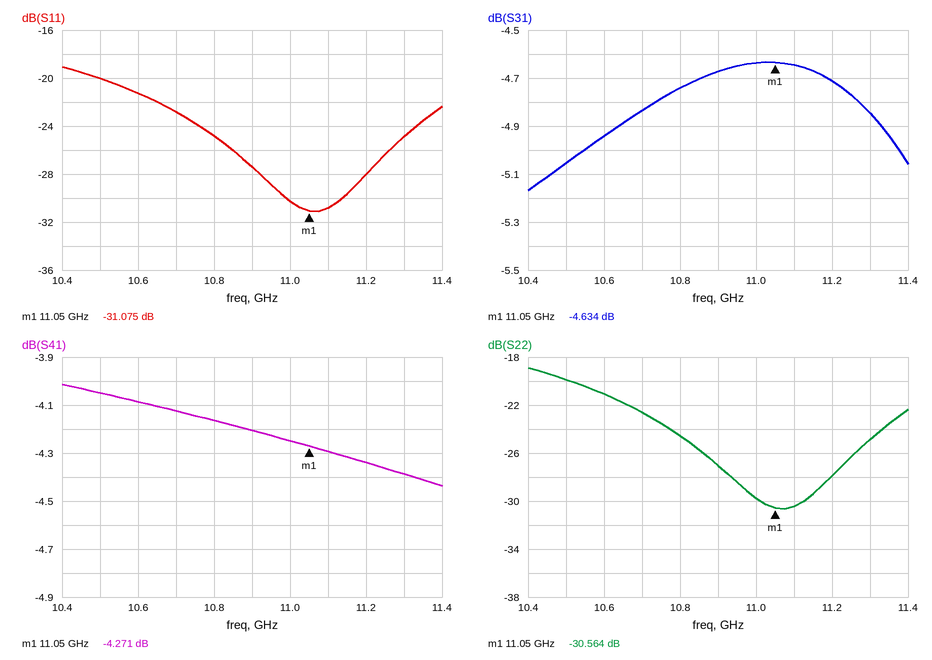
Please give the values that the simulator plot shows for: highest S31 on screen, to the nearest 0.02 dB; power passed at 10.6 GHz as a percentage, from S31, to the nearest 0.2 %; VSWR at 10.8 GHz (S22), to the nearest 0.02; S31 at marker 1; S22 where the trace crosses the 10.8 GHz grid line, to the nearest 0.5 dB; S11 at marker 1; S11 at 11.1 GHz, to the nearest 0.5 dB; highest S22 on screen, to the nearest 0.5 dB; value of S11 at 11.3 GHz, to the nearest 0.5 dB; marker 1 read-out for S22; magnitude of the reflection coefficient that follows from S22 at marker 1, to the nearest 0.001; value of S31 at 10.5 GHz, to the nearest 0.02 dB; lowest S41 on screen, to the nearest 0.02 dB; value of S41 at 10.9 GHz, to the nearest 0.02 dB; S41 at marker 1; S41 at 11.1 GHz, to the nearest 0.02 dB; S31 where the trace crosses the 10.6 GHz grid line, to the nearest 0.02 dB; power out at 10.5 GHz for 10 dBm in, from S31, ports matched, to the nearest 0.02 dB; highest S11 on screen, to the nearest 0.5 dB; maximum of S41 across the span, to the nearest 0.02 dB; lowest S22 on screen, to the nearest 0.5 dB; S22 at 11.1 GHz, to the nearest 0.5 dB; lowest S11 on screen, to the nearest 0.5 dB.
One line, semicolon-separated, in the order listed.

-4.64 dB; 32.0 %; 1.12; -4.634 dB; -24.5 dB; -31.075 dB; -31.0 dB; -19.0 dB; -25.0 dB; -30.564 dB; 0.030; -5.06 dB; -4.44 dB; -4.20 dB; -4.271 dB; -4.30 dB; -4.94 dB; 4.94 dBm; -19.0 dB; -4.02 dB; -30.5 dB; -30.5 dB; -31.0 dB
